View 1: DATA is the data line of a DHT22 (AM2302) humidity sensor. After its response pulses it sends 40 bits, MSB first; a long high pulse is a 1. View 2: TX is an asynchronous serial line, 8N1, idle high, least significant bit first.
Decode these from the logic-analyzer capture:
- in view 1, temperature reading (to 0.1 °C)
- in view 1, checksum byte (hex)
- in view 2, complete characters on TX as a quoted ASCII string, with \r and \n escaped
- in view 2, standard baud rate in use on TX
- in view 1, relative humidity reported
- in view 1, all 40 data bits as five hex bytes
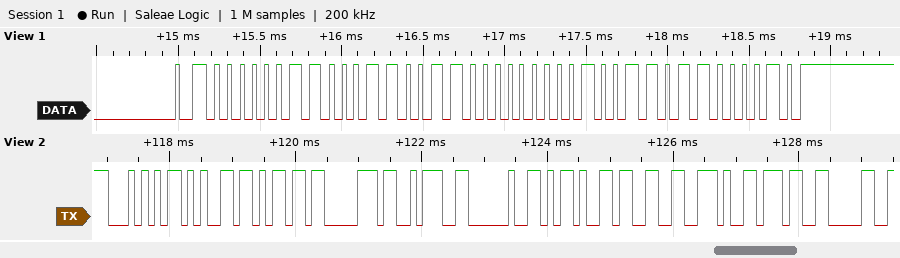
-3.8 °C
0xC2
"Temp: -3.70"
9600 baud
79.3 %
03 19 80 26 C2
